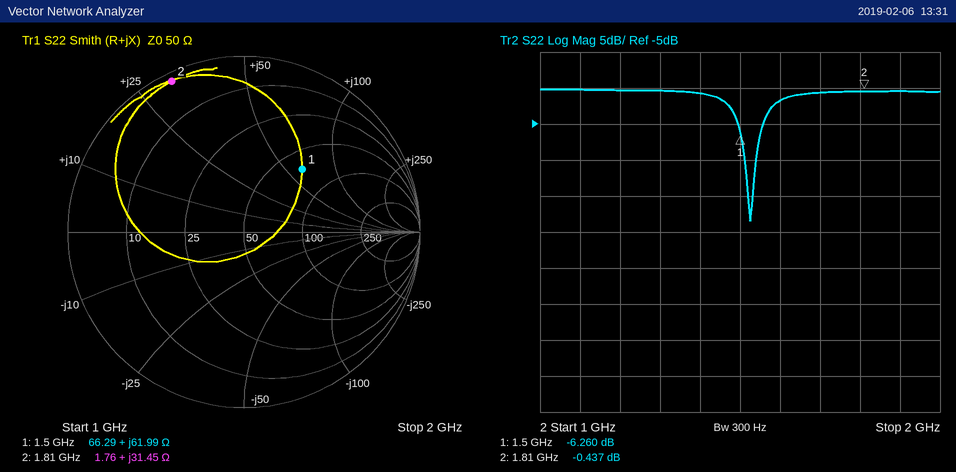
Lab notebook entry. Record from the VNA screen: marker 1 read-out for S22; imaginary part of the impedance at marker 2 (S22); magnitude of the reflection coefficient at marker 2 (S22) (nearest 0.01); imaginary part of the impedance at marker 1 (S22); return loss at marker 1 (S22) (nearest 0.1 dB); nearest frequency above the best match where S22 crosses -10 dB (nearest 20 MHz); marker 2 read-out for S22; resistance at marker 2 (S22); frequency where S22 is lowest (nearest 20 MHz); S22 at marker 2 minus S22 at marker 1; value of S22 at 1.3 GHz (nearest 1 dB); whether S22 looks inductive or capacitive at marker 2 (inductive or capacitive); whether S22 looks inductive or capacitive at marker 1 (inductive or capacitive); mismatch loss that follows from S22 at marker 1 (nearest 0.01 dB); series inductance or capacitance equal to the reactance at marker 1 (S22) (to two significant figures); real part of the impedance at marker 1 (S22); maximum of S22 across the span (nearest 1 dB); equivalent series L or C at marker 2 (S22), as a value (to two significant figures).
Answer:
-6.260 dB
+31.45 Ω
0.95
+61.99 Ω
6.3 dB
1.54 GHz
-0.437 dB
1.76 Ω
1.52 GHz
5.823 dB
0 dB
inductive
inductive
1.17 dB
6.6 nH
66.29 Ω
0 dB
2.8 nH
